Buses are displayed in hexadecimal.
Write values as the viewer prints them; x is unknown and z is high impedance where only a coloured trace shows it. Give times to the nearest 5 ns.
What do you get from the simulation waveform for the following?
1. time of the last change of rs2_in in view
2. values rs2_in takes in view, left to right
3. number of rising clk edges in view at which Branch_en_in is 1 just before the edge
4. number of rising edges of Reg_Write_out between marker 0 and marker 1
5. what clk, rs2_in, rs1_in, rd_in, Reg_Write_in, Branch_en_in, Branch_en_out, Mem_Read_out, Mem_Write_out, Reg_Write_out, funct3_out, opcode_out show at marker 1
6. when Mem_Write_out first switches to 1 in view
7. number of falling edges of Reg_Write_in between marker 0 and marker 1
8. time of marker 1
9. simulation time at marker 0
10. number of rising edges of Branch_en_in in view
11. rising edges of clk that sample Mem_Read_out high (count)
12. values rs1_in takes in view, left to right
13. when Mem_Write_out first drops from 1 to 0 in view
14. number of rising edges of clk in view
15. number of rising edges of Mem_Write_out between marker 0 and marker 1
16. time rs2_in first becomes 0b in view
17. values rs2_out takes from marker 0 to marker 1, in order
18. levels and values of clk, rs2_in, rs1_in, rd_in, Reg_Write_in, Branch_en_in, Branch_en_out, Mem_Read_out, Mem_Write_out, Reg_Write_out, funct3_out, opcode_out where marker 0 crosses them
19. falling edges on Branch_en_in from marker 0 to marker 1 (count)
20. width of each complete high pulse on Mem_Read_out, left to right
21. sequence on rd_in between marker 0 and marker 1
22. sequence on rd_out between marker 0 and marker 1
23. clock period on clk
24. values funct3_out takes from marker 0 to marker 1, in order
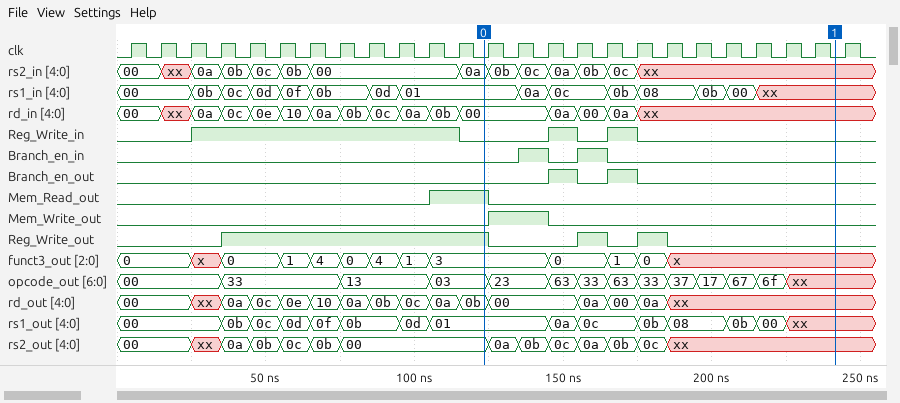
175 ns
00, xx, 0a, 0b, 0c, 0b, 00, 0a, 0b, 0c, 0a, 0b, 0c, xx
2
2
clk=0, rs2_in=xx, rs1_in=xx, rd_in=xx, Reg_Write_in=0, Branch_en_in=0, Branch_en_out=0, Mem_Read_out=0, Mem_Write_out=0, Reg_Write_out=0, funct3_out=x, opcode_out=xx
125 ns
2
240 ns
125 ns
2
2
00, 0b, 0c, 0d, 0f, 0b, 0d, 01, 0a, 0c, 0b, 08, 0b, 00, xx
145 ns
25
1
35 ns
00, 0a, 0b, 0c, 0a, 0b, 0c, xx
clk=0, rs2_in=0a, rs1_in=01, rd_in=00, Reg_Write_in=0, Branch_en_in=0, Branch_en_out=0, Mem_Read_out=1, Mem_Write_out=0, Reg_Write_out=1, funct3_out=3, opcode_out=03
2
20 ns
00, 0a, 00, 0a, xx
0b, 00, 0a, 00, 0a, xx
10 ns
3, 0, 1, 0, x
